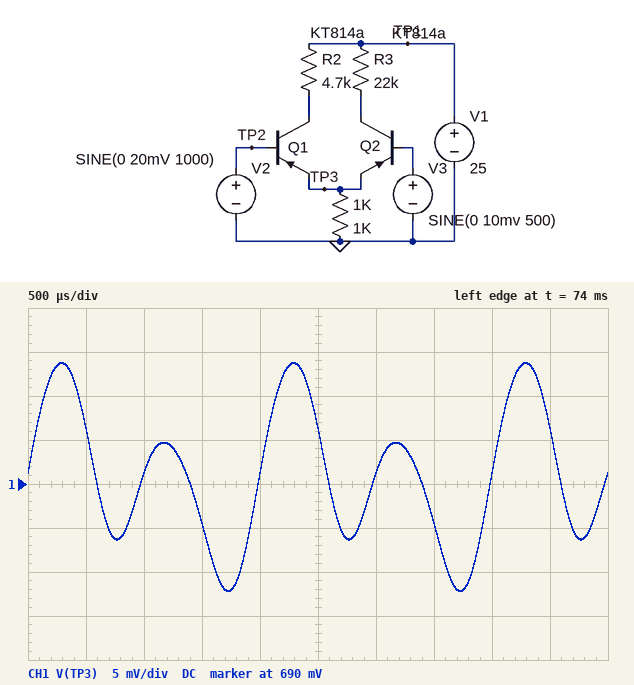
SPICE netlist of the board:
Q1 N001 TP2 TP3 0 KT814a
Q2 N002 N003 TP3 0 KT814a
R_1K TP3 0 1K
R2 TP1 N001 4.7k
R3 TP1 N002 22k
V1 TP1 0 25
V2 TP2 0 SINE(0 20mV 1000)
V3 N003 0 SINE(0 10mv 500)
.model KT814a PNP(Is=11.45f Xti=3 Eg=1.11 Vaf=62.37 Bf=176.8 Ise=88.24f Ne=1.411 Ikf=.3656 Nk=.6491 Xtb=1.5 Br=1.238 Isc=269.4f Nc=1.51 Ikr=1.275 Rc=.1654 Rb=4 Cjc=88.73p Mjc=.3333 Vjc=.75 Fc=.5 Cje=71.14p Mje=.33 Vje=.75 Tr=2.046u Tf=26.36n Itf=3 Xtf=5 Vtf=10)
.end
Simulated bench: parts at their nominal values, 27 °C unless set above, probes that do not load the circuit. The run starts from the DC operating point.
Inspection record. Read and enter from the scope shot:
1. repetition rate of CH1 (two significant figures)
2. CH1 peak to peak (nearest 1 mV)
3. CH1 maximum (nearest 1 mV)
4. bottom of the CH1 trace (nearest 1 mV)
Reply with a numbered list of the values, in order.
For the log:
1. 1.0 kHz
2. 26 mV
3. 704 mV
4. 678 mV
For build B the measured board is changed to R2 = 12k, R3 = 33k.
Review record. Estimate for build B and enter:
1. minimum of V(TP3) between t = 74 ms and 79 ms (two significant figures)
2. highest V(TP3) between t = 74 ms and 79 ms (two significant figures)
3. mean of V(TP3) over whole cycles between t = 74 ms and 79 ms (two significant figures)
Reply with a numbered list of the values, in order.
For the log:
1. 640 mV
2. 670 mV
3. 650 mV
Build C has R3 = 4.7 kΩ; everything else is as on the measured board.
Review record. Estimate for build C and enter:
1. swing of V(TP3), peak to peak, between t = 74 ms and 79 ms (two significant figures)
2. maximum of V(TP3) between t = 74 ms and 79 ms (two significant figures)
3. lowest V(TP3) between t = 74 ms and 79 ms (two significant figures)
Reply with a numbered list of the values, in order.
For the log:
1. 27 mV
2. 730 mV
3. 700 mV
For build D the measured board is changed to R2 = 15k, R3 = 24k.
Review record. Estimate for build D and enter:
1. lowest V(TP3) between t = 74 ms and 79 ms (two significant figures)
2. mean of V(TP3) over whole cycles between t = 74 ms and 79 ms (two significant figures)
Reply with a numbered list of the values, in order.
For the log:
1. 640 mV
2. 650 mV
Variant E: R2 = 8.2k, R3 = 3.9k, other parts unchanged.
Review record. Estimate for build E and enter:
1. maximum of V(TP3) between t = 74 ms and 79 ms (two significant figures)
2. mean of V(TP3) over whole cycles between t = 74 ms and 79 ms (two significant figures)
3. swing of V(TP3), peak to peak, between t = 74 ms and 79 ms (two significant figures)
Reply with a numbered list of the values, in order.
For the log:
1. 720 mV
2. 710 mV
3. 28 mV
